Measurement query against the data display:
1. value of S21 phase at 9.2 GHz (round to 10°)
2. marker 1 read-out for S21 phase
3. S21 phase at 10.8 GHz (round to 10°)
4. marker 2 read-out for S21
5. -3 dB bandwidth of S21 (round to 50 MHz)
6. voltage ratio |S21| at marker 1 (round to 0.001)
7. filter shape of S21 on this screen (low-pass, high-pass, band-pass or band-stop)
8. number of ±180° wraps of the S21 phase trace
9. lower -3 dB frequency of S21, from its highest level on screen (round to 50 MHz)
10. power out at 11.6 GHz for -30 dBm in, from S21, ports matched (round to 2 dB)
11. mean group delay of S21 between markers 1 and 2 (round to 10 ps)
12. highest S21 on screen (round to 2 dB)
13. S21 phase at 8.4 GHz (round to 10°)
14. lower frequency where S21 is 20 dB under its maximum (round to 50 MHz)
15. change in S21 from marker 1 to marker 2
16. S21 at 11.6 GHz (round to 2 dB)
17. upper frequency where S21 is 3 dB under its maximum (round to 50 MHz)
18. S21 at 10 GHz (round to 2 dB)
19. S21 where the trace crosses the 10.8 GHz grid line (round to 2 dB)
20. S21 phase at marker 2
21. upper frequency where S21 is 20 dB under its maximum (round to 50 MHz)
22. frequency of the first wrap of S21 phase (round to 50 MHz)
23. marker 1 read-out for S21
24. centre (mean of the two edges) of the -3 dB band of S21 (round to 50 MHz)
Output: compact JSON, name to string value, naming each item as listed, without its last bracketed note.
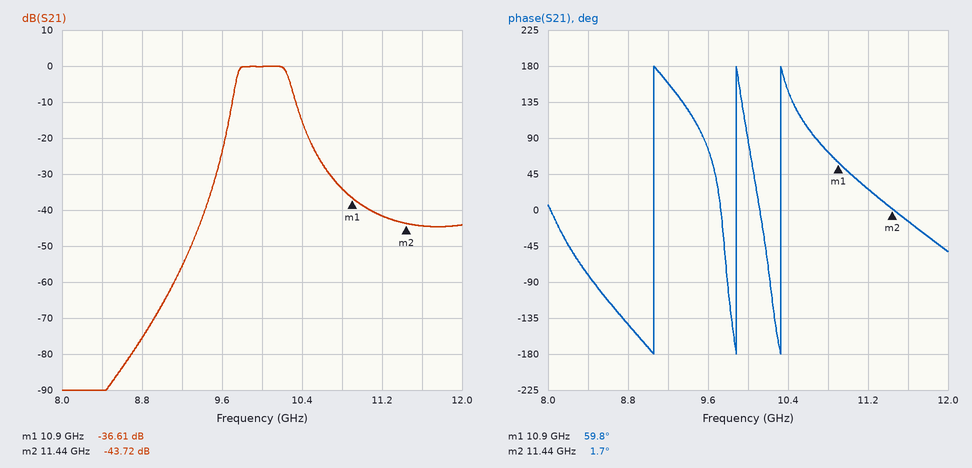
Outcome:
{"value of S21 phase at 9.2 GHz": "160°", "marker 1 read-out for S21 phase": "59.8°", "S21 phase at 10.8 GHz": "70°", "marker 2 read-out for S21": "-43.72 dB", "-3 dB bandwidth of S21": "500 MHz", "voltage ratio |S21| at marker 1": "0.015", "filter shape of S21 on this screen": "band-pass", "number of ±180° wraps of the S21 phase trace": "3", "lower -3 dB frequency of S21, from its highest level on screen": "9.75 GHz", "power out at 11.6 GHz for -30 dBm in, from S21, ports matched": "-74 dBm", "mean group delay of S21 between markers 1 and 2": "300 ps", "highest S21 on screen": "0 dB", "S21 phase at 8.4 GHz": "-80°", "lower frequency where S21 is 20 dB under its maximum": "9.65 GHz", "change in S21 from marker 1 to marker 2": "-7.11 dB", "S21 at 11.6 GHz": "-44 dB", "upper frequency where S21 is 3 dB under its maximum": "10.25 GHz", "S21 at 10 GHz": "0 dB", "S21 where the trace crosses the 10.8 GHz grid line": "-34 dB", "S21 phase at marker 2": "1.7°", "upper frequency where S21 is 20 dB under its maximum": "10.45 GHz", "frequency of the first wrap of S21 phase": "9.05 GHz", "marker 1 read-out for S21": "-36.61 dB", "centre (mean of the two edges) of the -3 dB band of S21": "10.00 GHz"}
